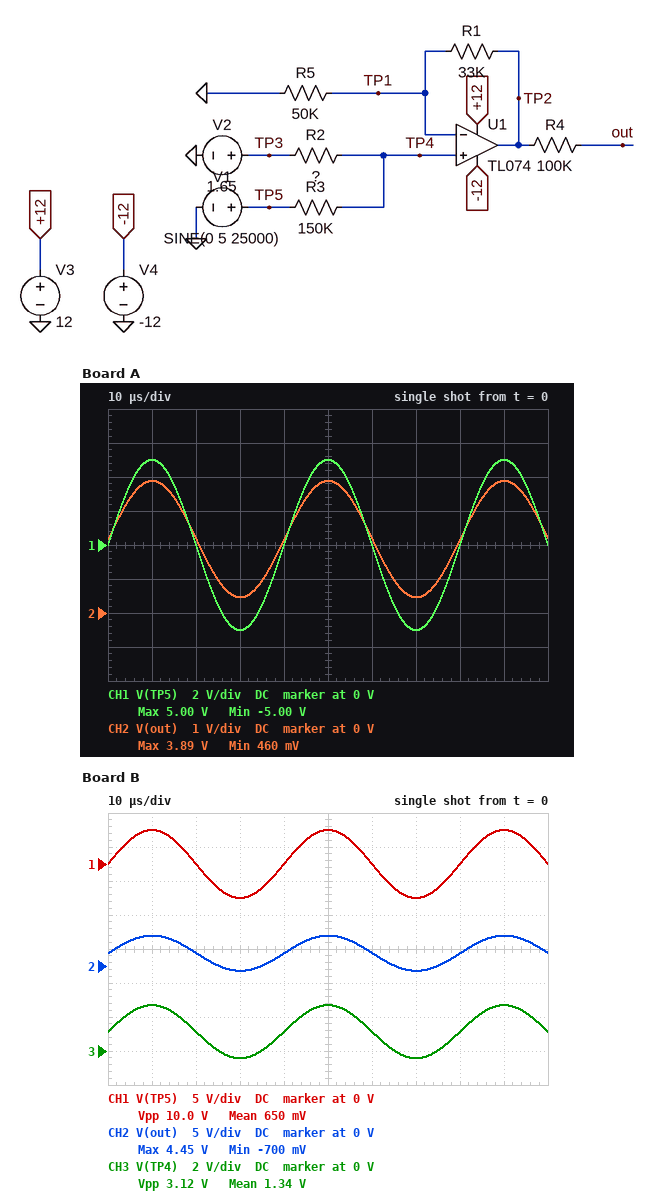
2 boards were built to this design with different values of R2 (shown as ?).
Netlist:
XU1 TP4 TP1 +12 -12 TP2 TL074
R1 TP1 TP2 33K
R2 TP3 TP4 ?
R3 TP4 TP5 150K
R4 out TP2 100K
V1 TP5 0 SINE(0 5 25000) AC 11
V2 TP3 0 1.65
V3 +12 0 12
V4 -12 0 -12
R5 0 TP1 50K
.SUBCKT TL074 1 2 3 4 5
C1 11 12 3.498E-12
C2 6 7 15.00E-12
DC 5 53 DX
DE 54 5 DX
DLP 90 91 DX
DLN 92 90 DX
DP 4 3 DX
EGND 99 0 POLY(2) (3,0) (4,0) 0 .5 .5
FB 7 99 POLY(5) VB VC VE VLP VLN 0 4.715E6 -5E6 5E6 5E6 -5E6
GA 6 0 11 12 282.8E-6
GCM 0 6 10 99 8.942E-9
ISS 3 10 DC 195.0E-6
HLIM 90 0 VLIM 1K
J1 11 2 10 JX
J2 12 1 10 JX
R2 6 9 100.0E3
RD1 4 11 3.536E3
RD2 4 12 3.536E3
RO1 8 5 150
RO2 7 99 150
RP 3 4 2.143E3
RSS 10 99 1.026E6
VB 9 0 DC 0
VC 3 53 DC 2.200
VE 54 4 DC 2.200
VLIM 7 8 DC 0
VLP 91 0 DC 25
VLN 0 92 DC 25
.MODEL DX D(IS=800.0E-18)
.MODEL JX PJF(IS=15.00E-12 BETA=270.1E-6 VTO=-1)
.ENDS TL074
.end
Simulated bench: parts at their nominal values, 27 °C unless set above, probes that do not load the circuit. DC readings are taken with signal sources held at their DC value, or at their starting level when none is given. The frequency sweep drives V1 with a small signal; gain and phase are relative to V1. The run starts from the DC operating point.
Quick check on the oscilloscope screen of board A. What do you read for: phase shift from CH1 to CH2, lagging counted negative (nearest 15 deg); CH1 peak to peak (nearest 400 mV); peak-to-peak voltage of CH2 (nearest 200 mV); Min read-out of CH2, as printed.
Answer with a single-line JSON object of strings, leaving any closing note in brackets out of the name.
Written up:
{"phase shift from CH1 to CH2, lagging counted negative": "0 deg", "CH1 peak to peak": "10.0 V", "peak-to-peak voltage of CH2": "3.4 V", "Min read-out of CH2, as printed": "460 mV"}
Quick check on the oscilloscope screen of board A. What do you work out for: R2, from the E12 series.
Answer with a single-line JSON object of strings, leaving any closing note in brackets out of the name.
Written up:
{"R2, from the E12 series": "39 kΩ"}
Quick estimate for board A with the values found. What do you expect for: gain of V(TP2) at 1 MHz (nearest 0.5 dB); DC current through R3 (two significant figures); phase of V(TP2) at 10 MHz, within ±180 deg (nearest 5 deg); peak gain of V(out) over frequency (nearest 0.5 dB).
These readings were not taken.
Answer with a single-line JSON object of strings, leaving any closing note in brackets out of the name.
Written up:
{"gain of V(TP2) at 1 MHz": "-9.5 dB", "DC current through R3": "8.7 µA", "phase of V(TP2) at 10 MHz, within ±180 deg": "-145 deg", "peak gain of V(out) over frequency": "-9.5 dB"}
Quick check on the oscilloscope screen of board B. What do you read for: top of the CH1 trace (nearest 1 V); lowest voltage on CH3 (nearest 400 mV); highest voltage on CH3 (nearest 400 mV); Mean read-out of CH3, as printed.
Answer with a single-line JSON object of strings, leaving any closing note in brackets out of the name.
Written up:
{"top of the CH1 trace": "5 V", "lowest voltage on CH3": "-400 mV", "highest voltage on CH3": "2.8 V", "Mean read-out of CH3, as printed": "1.34 V"}
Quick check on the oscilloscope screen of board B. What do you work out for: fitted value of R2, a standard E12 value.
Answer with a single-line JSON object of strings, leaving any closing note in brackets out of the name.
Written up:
{"fitted value of R2, a standard E12 value": "68 kΩ"}
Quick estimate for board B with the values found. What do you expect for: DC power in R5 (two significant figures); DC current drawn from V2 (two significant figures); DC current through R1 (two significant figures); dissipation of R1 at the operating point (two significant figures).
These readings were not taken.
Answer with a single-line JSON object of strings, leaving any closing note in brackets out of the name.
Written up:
{"DC power in R5": "26 µW", "DC current drawn from V2": "7.6 µA", "DC current through R1": "23 µA", "dissipation of R1 at the operating point": "17 µW"}
